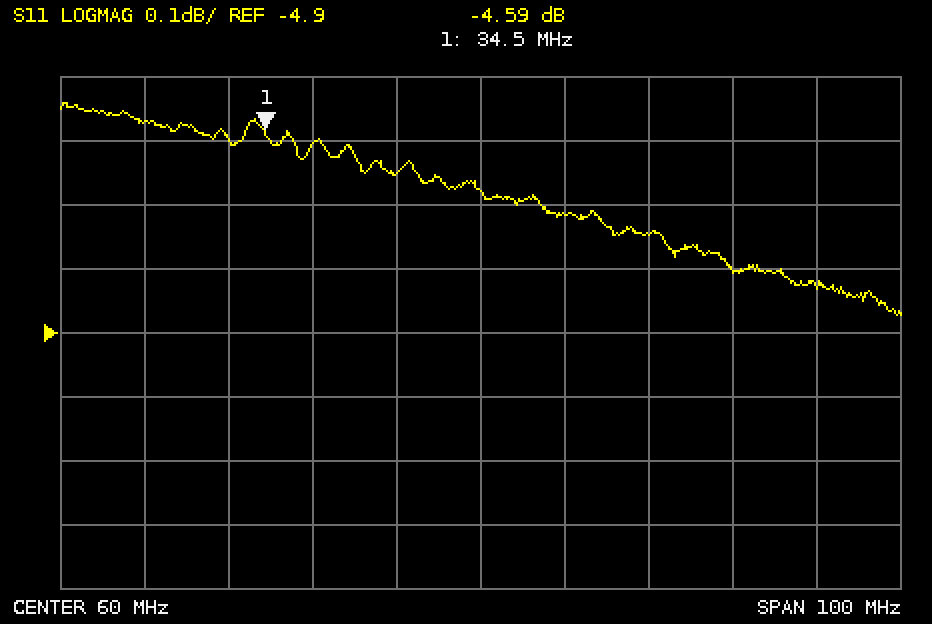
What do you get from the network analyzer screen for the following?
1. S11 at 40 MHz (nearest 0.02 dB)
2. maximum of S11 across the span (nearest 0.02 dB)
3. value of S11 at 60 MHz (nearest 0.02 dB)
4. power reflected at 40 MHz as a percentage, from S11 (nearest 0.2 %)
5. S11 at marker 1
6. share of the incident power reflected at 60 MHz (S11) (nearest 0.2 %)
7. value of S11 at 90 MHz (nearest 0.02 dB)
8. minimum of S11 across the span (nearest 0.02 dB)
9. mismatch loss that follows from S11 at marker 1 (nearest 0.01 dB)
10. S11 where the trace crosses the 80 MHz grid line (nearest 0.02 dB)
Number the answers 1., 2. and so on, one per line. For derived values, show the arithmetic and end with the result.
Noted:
1. -4.60 dB
2. -4.54 dB
3. -4.68 dB
4. 10^(-4.6/10) ≈ 34.7 %, so 34.6 % to the nearest 0.2 %
5. -4.59 dB
6. 10^(-4.68/10) ≈ 34.0 %
7. -4.80 dB
8. -4.88 dB
9. −10 log10(1 − 10^(-4.59/10)) ≈ 1.85 dB
10. -4.74 dB
